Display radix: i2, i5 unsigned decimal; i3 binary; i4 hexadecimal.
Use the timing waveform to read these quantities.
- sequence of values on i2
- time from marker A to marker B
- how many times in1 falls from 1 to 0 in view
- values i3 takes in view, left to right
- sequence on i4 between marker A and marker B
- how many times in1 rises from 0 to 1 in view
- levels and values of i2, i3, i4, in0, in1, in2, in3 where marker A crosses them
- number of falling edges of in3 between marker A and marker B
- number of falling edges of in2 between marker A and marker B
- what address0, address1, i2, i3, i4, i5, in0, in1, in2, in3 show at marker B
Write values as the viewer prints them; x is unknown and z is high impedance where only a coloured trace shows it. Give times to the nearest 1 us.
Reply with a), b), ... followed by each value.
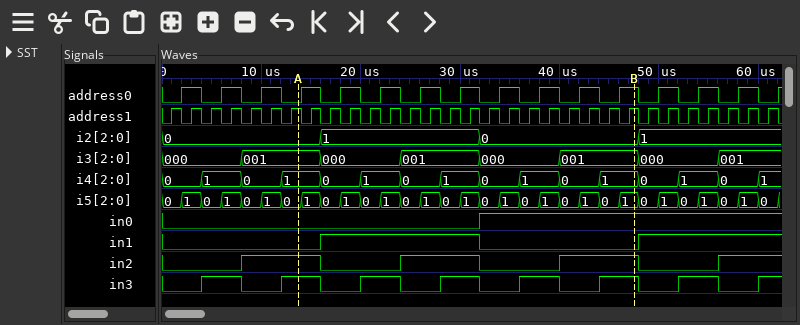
a) 0, 1, 0, 1
b) 34 us
c) 1
d) 000, 001, 000, 001, 000, 001, 000, 001
e) 1, 0, 1, 0, 1, 0, 1, 0, 1
f) 2
g) i2=0, i3=001, i4=1, in0=0, in1=0, in2=1, in3=1
h) 4
i) 2
j) address0=1, address1=1, i2=0, i3=001, i4=1, i5=1, in0=1, in1=0, in2=1, in3=1
